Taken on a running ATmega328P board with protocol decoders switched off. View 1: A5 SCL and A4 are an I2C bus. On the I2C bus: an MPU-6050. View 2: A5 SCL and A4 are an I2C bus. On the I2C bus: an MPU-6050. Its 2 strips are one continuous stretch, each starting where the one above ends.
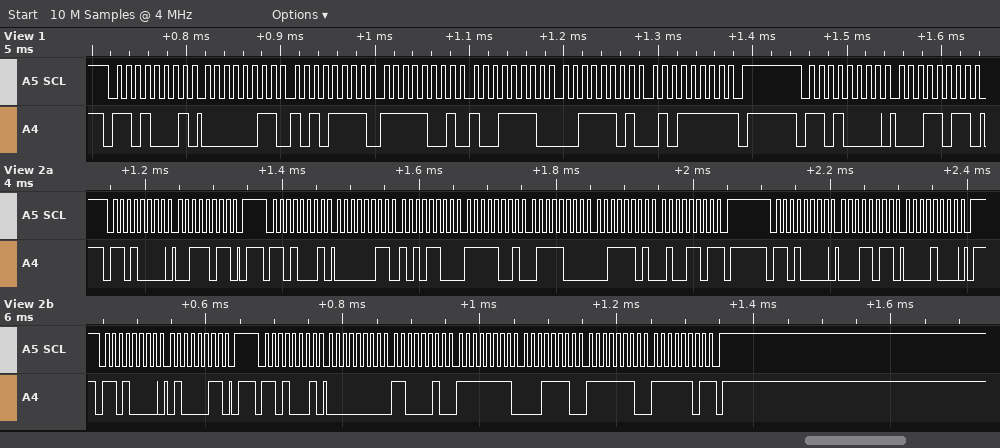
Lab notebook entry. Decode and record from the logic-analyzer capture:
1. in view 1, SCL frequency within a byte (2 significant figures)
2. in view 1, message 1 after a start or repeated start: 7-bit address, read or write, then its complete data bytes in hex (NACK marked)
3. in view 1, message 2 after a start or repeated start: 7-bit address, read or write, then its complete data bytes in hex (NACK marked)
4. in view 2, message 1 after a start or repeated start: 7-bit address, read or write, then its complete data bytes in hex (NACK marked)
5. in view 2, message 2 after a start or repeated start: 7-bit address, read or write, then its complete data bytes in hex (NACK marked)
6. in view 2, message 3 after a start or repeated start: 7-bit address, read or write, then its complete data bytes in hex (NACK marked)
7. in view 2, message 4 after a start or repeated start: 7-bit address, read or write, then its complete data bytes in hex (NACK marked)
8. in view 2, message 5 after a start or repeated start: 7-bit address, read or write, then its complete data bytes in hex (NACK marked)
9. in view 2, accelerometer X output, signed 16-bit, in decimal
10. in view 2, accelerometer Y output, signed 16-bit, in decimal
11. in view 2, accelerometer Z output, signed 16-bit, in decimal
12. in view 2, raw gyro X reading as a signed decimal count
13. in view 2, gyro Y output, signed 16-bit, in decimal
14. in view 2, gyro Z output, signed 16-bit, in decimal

100 kHz
0x68 read: 03 AF F9 9E 3D 5F NACK
0x68 write: 1B
0x68 write: 3B
0x68 read: 03 AC F9 78 3D 4D NACK
0x68 write: 1B 08
0x68 write: 43
0x68 read: 00 C2 FF 1E FE FD NACK
940
-1672
15693
194
-226
-259
